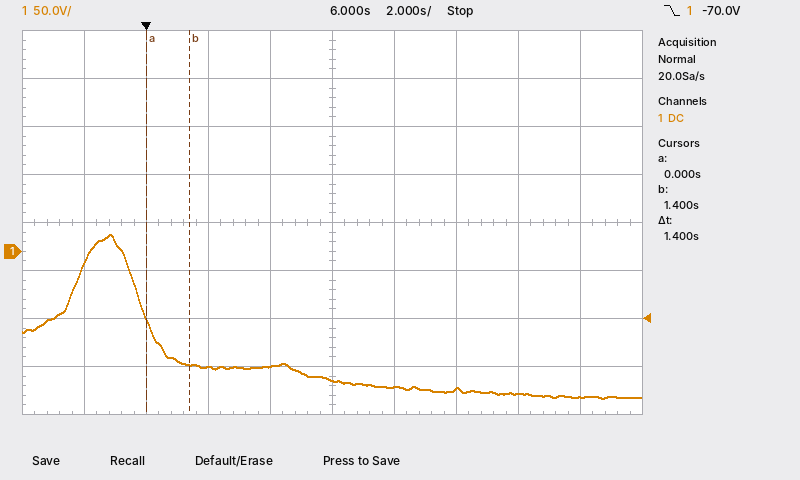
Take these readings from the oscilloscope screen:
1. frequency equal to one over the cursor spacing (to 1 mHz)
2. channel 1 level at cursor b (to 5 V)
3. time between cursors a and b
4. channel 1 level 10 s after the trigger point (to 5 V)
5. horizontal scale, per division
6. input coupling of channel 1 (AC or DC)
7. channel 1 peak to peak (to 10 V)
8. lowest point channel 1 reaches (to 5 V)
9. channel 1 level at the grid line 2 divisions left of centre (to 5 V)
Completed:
714 mHz
-120 V
1.4 s
-145 V
2 s
DC
170 V
-155 V
-120 V
